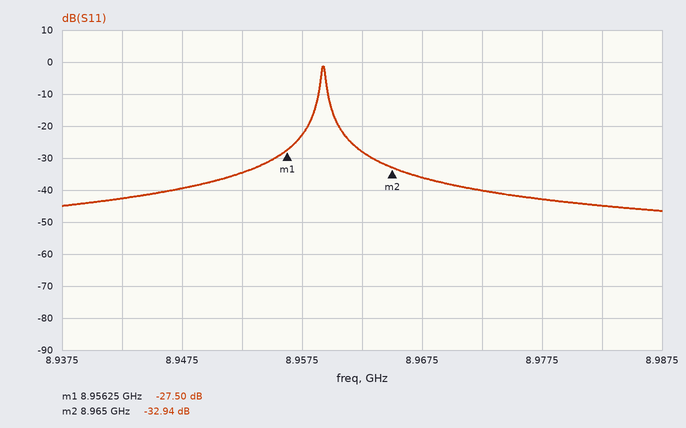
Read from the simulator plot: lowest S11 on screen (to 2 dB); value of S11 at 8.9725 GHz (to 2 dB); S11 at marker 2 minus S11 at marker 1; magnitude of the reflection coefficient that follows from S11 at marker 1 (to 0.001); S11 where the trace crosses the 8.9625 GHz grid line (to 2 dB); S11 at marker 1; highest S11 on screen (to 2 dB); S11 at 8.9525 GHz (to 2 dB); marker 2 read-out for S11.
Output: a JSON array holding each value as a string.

["-46 dB", "-40 dB", "-5.44 dB", "0.042", "-28 dB", "-27.50 dB", "-2 dB", "-34 dB", "-32.94 dB"]
